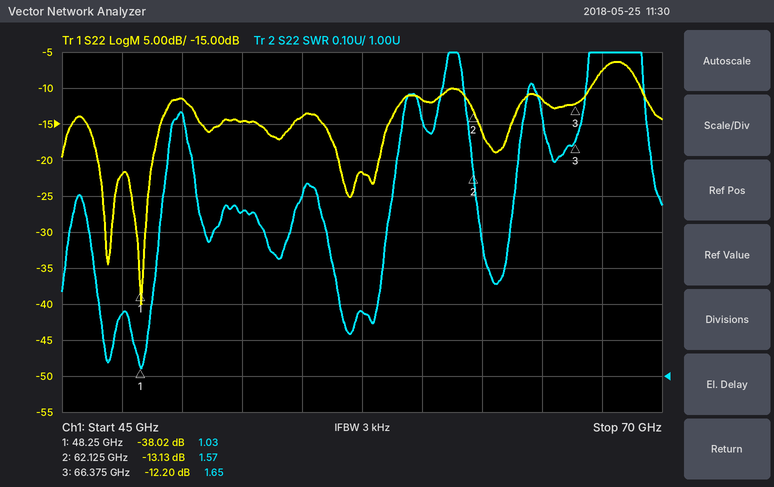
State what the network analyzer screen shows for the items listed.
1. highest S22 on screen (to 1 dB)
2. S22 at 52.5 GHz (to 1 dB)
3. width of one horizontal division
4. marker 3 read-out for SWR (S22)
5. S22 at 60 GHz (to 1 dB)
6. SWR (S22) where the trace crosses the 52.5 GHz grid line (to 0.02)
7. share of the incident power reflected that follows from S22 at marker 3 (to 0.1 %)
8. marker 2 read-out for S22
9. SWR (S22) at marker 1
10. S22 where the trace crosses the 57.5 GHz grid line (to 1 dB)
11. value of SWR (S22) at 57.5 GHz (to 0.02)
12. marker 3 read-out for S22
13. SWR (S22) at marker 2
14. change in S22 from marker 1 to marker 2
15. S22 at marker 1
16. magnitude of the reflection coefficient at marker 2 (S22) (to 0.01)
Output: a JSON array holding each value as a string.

["-6 dB", "-15 dB", "2.5 GHz", "1.65", "-12 dB", "1.46", "6.0 %", "-13.13 dB", "1.03", "-22 dB", "1.18", "-12.20 dB", "1.57", "24.89 dB", "-38.02 dB", "0.22"]
